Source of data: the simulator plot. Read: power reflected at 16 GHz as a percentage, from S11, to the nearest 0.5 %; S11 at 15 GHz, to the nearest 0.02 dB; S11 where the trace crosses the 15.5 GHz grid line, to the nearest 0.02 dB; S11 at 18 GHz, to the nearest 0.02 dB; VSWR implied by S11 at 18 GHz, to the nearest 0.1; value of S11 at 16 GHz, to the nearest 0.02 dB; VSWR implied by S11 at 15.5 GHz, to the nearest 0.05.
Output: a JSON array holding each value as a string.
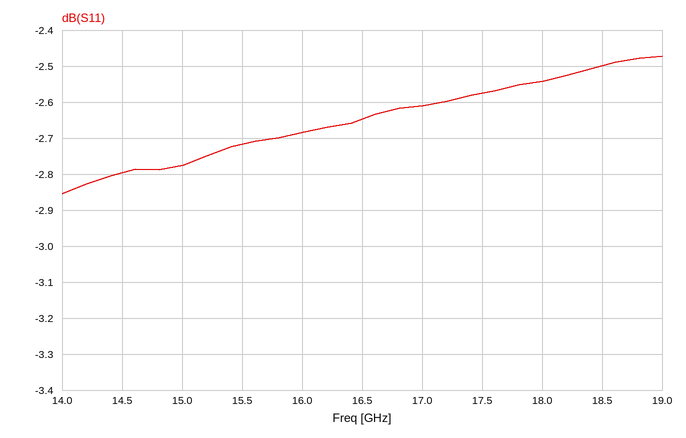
["54.0 %", "-2.78 dB", "-2.72 dB", "-2.54 dB", "6.9", "-2.68 dB", "6.45"]
